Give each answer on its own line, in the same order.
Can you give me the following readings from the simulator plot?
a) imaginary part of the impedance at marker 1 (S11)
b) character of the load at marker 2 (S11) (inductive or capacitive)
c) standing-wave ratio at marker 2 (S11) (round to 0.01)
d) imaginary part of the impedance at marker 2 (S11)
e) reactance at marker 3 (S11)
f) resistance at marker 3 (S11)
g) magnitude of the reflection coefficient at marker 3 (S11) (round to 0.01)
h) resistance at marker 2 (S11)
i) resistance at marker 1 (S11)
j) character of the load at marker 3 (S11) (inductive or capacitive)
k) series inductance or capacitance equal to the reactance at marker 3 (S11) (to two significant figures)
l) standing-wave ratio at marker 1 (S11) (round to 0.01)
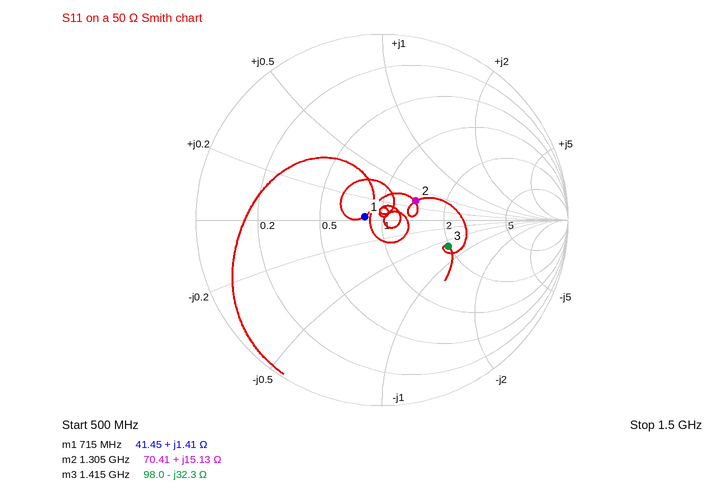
+1.41 Ω
inductive
1.53
+15.13 Ω
-32.3 Ω
98.0 Ω
0.38
70.41 Ω
41.45 Ω
capacitive
3.5 pF
1.21
